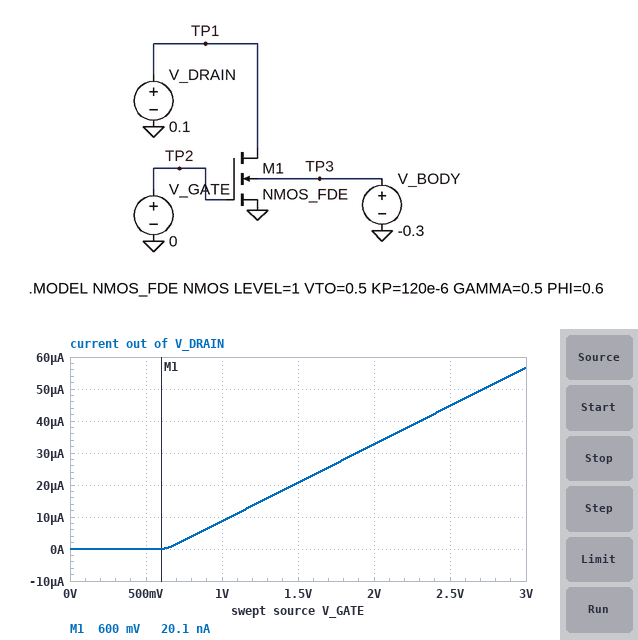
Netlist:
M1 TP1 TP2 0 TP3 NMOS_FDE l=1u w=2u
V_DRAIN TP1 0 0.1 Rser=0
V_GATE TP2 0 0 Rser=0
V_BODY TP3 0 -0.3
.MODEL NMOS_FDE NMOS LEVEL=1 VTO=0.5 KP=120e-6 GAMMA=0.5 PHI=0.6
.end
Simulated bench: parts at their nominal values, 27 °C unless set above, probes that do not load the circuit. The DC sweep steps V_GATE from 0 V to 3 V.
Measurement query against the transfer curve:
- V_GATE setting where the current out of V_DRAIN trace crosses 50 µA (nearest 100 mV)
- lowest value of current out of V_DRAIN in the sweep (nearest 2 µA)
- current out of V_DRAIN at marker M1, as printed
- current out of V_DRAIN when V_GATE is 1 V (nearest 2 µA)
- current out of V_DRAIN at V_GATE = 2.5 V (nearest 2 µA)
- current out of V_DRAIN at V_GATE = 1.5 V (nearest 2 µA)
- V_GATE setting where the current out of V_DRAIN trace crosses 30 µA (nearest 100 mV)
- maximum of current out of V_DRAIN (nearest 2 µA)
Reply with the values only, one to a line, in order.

2.7 V
0 A
20.1 nA
8 µA
44 µA
20 µA
1.9 V
56 µA
